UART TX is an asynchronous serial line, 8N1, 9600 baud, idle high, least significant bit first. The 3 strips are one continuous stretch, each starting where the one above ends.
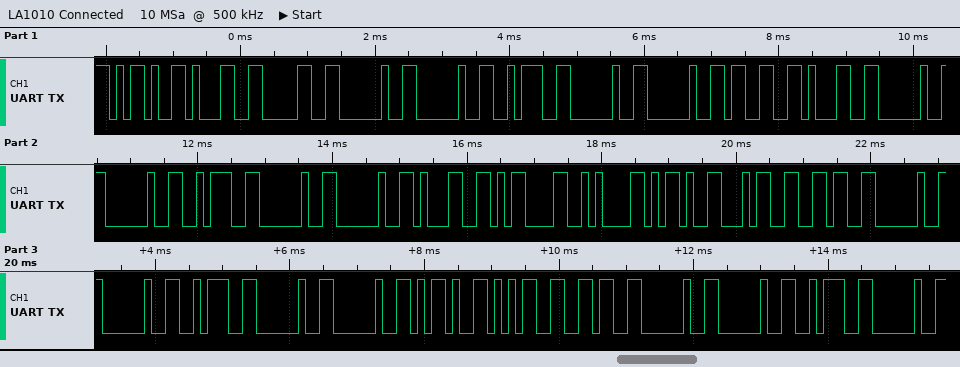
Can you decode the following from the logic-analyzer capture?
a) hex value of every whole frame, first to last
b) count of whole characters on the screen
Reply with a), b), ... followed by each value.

a) 2D 31 30 20 20 3A 20 20 33 31 20 20 3A 20 20 31 0D 0A 2D 34 36 20 20 3A 20 20 2D 35 36 20 20 3A 20
b) 33
